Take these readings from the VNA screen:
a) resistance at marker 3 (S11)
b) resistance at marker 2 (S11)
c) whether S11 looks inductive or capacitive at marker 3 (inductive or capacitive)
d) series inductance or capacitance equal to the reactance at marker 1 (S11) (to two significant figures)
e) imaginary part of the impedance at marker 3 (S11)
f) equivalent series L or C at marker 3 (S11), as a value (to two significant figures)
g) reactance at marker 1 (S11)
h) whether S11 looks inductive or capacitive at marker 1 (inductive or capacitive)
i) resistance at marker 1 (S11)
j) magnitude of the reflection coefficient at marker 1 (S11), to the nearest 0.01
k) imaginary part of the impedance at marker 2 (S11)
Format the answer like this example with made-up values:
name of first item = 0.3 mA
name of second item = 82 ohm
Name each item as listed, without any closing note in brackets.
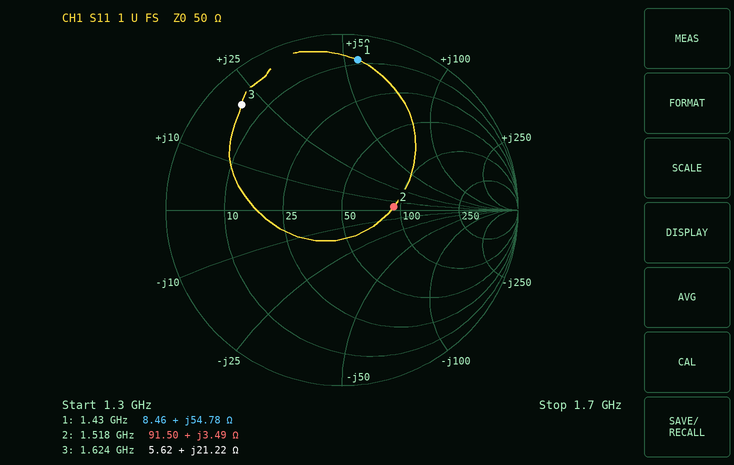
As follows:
resistance at marker 3 = 5.62 Ω
resistance at marker 2 = 91.50 Ω
whether S11 looks inductive or capacitive at marker 3 = inductive
series inductance or capacitance equal to the reactance at marker 1 (S11) = 6.1 nH
imaginary part of the impedance at marker 3 = +21.22 Ω
equivalent series L or C at marker 3 (S11), as a value = 2.1 nH
reactance at marker 1 = +54.78 Ω
whether S11 looks inductive or capacitive at marker 1 = inductive
resistance at marker 1 = 8.46 Ω
magnitude of the reflection coefficient at marker 1 (S11), to the nearest 0.01 = 0.86
imaginary part of the impedance at marker 2 = +3.49 Ω
